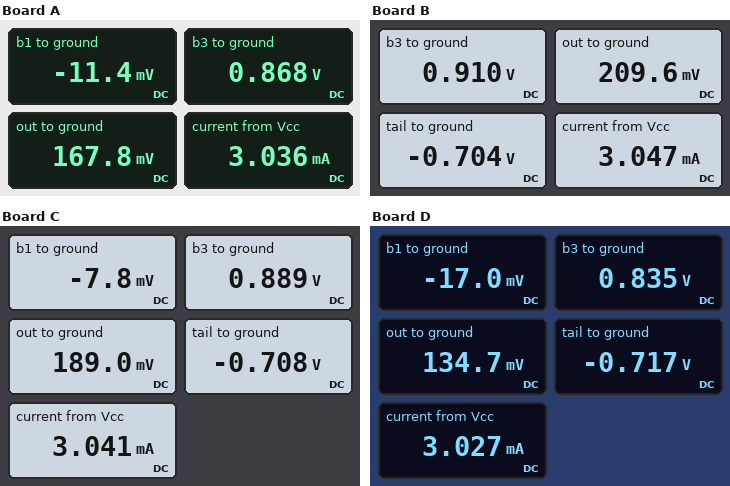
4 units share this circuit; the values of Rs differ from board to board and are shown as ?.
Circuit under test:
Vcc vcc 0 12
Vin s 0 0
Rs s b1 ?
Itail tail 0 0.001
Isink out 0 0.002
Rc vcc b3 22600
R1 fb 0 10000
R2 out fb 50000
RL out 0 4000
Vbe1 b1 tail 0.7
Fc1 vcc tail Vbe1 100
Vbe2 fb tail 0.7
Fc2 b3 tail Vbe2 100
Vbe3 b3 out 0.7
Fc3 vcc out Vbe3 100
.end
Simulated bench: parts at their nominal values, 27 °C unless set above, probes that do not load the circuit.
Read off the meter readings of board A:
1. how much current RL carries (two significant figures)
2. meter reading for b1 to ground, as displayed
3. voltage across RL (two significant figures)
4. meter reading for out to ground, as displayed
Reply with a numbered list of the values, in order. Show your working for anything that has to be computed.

1. (167.8 mV) / 4 kΩ = 42 µA
2. -11.4 mV
3. 167.8 mV = 170 mV
4. 167.8 mV
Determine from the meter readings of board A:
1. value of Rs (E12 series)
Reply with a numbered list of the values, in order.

1. 2.2 kΩ
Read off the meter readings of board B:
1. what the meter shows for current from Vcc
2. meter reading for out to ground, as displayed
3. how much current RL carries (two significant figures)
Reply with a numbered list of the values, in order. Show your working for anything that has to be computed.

1. 3.047 mA
2. 209.6 mV
3. (209.6 mV) / 4 kΩ = 52 µA
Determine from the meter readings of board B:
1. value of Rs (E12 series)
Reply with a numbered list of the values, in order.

1. 820 Ω
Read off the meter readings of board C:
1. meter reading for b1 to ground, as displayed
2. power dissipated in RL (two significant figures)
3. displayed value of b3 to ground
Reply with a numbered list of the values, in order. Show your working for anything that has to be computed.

1. -7.8 mV
2. (189 mV)^2 / 4 kΩ = 8.9 µW
3. 0.889 V
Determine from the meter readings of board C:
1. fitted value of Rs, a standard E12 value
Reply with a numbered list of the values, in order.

1. 1.5 kΩ
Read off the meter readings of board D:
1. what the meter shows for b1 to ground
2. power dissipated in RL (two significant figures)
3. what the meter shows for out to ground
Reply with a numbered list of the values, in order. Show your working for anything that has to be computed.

1. -17.0 mV
2. (134.7 mV)^2 / 4 kΩ = 4.5 µW
3. 134.7 mV
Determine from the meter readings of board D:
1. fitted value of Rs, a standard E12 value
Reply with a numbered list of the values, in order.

1. 3.3 kΩ
